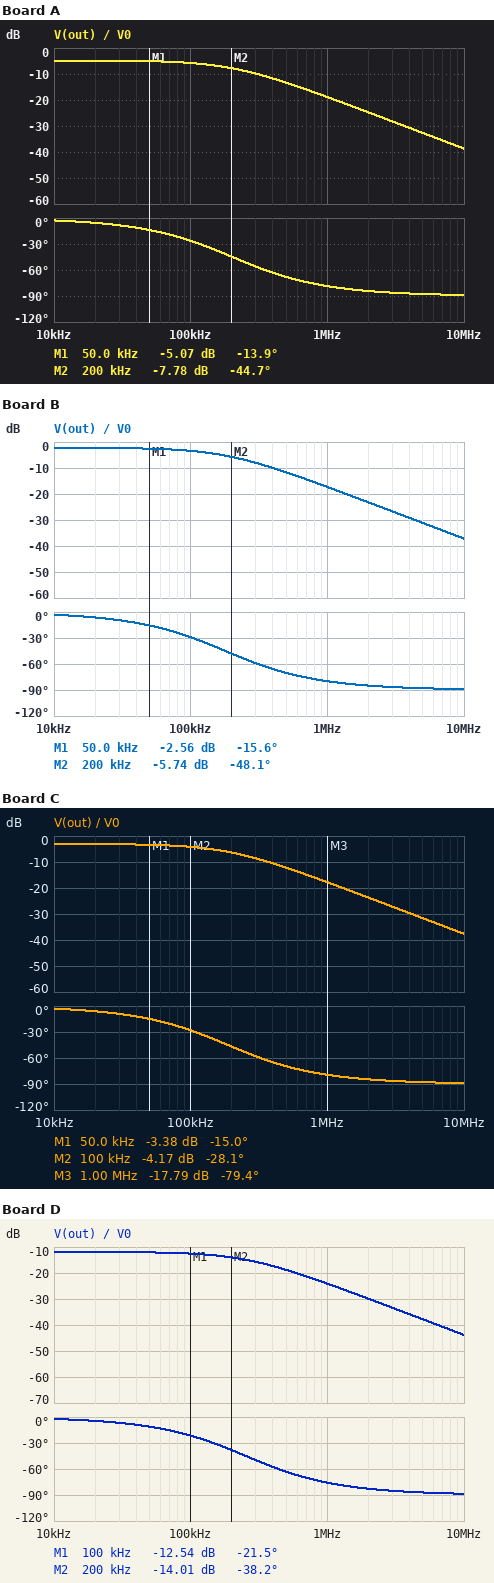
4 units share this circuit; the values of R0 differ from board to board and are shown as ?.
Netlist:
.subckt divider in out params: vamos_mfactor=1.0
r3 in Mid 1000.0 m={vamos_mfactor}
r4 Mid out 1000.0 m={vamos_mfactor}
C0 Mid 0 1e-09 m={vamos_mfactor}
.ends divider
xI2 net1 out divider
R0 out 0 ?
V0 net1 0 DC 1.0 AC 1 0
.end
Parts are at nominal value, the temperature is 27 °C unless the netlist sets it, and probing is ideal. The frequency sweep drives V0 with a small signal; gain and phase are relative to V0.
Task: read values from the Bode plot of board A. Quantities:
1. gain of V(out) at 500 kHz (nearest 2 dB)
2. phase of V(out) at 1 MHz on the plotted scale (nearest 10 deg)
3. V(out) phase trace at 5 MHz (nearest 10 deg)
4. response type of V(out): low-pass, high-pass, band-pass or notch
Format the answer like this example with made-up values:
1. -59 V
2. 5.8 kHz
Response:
1. -14 dB
2. -80 deg
3. -90 deg
4. low-pass
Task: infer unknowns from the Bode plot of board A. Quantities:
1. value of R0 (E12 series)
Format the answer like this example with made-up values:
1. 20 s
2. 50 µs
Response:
1. 2.7 kΩ
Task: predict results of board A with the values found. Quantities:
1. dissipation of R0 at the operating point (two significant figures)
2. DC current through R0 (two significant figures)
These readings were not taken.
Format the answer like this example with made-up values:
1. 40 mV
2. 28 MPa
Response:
1. 120 µW
2. 210 µA
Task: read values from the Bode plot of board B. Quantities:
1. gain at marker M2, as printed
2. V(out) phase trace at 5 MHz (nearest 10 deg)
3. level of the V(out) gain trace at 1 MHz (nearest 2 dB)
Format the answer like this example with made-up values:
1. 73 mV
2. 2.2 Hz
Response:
1. -5.74 dB
2. -90 deg
3. -18 dB
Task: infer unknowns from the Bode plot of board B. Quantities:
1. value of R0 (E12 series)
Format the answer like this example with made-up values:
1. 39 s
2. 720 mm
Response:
1. 6.8 kΩ
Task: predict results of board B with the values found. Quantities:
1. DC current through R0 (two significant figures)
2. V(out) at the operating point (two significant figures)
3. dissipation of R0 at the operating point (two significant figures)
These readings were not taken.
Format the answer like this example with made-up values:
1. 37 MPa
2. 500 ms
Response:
1. 110 µA
2. 770 mV
3. 88 µW
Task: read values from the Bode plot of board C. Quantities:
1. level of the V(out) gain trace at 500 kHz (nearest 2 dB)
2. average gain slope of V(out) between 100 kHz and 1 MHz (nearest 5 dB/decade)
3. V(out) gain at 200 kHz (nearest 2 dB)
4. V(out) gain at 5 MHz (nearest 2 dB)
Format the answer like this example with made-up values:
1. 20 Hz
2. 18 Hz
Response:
1. -12 dB
2. -15 dB/decade
3. -6 dB
4. -32 dB
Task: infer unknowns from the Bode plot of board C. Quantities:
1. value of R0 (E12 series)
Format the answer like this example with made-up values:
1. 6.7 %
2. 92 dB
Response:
1. 4.7 kΩ
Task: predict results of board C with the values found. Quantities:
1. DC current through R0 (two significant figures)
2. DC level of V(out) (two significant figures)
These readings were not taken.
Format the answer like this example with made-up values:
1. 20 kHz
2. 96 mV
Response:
1. 150 µA
2. 700 mV
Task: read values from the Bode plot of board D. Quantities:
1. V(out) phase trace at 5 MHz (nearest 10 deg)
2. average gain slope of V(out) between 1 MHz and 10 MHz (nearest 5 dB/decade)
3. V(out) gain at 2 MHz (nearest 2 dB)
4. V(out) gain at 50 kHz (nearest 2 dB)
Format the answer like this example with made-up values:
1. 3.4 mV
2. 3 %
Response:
1. -90 deg
2. -20 dB/decade
3. -30 dB
4. -12 dB
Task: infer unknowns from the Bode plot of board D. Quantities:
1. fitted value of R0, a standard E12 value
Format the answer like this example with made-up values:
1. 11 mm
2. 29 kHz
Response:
1. 680 Ω
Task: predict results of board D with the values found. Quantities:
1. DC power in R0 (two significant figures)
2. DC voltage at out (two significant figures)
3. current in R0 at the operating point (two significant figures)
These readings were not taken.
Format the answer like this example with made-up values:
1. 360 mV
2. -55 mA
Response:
1. 95 µW
2. 250 mV
3. 370 µA
